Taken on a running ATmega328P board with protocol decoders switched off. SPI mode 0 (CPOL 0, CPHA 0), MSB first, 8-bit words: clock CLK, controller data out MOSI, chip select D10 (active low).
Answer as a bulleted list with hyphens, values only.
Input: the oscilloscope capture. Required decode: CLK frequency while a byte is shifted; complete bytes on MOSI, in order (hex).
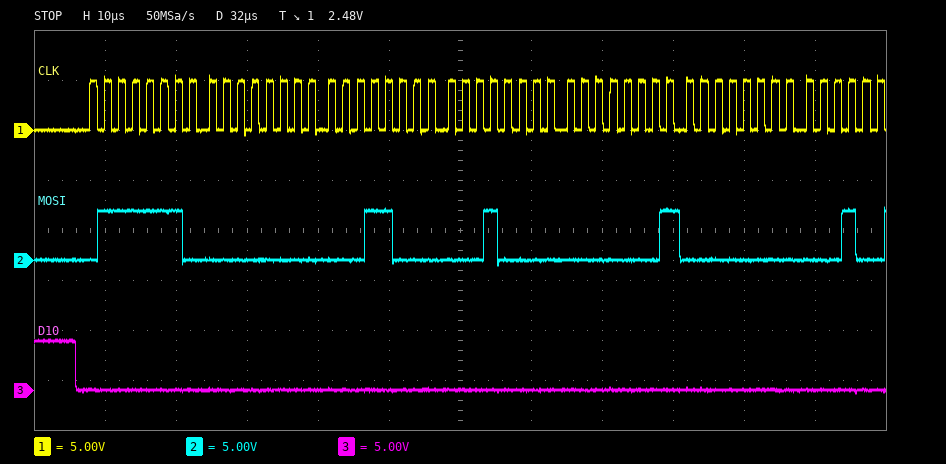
- 500 kHz
- 7E 00 18 10 01 00
